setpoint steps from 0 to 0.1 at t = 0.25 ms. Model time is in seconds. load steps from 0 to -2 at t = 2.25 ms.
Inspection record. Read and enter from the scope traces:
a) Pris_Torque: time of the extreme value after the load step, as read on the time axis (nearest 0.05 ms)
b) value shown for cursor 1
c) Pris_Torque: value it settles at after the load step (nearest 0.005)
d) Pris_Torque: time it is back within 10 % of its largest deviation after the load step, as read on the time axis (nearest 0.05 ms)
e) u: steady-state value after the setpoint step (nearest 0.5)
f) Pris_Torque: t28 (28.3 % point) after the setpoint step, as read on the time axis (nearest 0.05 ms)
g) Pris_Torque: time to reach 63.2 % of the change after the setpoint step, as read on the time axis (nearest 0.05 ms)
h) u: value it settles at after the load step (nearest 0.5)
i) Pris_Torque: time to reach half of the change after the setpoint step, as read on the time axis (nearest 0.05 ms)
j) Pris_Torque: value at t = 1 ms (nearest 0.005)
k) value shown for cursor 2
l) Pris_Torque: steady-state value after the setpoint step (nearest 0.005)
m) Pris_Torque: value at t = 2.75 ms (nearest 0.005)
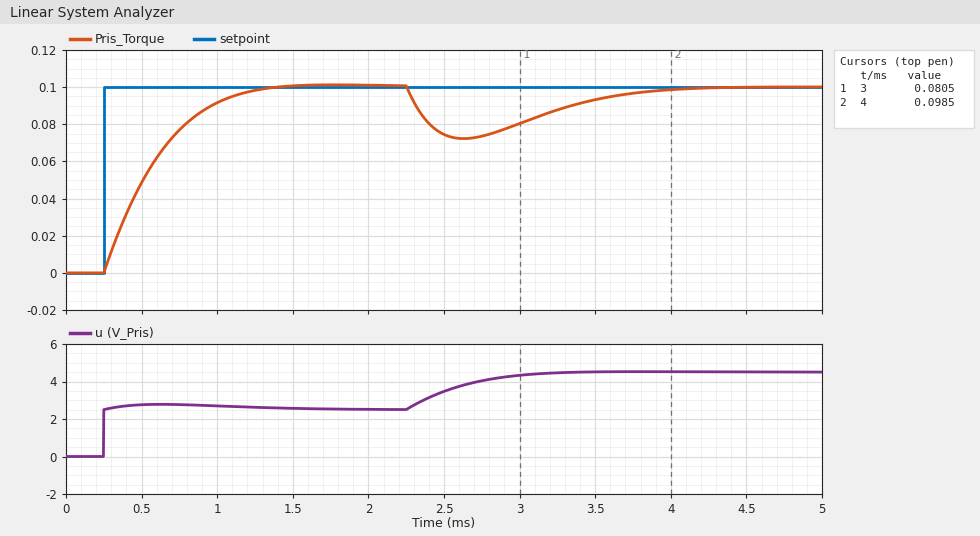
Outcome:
2.65 ms
0.0805
0.100
3.80 ms
2.5
0.40 ms
0.60 ms
4.5
0.50 ms
0.090
0.0985
0.100
0.075
